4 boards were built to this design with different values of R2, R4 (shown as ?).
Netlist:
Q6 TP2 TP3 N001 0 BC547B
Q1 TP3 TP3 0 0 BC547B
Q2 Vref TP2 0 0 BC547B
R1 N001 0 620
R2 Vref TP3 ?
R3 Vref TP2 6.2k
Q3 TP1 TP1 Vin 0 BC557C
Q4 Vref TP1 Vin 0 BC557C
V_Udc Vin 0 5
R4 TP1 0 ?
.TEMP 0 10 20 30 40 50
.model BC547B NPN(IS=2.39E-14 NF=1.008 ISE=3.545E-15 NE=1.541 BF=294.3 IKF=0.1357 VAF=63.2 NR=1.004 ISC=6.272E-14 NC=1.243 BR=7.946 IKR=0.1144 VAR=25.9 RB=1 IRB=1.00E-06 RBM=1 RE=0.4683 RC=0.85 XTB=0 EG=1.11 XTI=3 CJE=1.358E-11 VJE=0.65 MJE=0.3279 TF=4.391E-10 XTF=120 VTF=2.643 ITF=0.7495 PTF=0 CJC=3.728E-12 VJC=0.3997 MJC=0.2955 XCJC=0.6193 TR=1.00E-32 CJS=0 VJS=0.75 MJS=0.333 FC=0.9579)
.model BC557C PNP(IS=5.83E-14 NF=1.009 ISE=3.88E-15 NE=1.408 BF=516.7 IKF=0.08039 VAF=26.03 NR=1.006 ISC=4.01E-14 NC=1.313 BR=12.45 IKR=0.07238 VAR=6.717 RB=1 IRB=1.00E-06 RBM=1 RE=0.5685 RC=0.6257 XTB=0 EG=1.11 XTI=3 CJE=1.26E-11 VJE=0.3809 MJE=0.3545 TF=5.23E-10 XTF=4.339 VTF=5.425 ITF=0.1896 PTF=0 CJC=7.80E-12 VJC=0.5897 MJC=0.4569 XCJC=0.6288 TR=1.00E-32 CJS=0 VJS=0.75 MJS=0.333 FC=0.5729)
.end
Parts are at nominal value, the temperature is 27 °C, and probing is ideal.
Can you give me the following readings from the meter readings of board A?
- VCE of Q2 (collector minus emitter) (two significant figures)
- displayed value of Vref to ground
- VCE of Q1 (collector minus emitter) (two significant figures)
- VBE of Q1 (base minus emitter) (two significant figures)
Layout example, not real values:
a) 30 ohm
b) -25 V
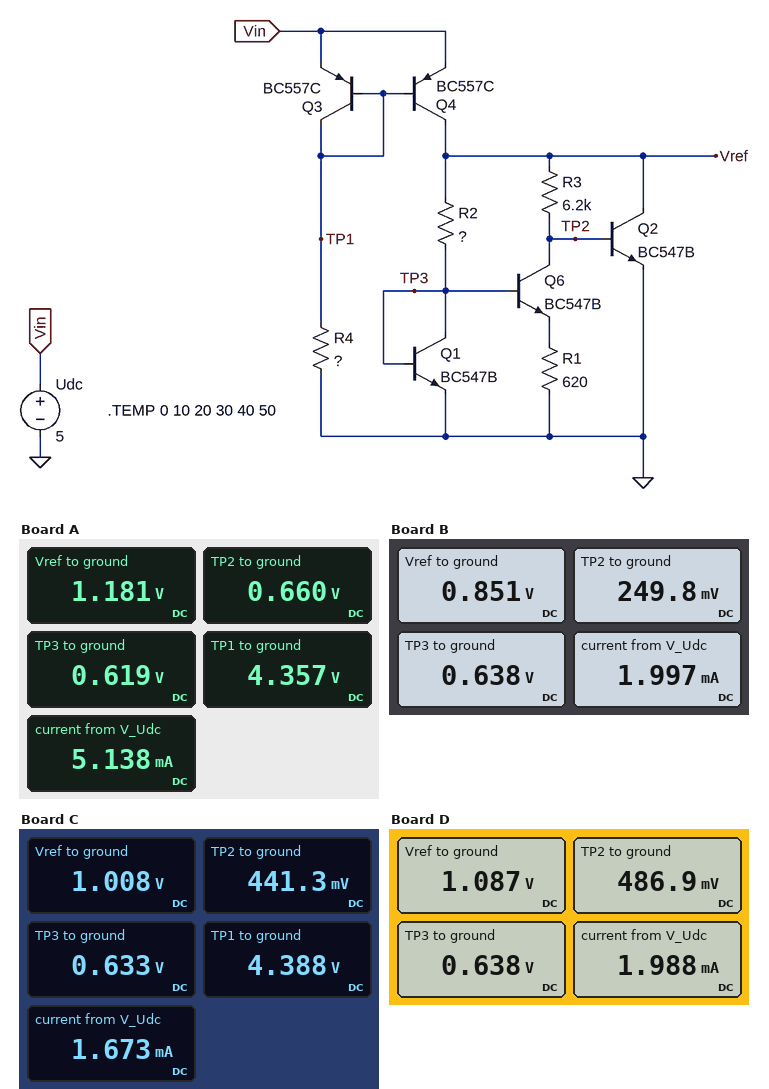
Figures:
a) 1.2 V
b) 1.181 V
c) 620 mV
d) 620 mV
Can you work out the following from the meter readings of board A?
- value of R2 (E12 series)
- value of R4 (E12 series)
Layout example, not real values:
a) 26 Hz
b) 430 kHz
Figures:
a) 1.2 kΩ
b) 1.8 kΩ
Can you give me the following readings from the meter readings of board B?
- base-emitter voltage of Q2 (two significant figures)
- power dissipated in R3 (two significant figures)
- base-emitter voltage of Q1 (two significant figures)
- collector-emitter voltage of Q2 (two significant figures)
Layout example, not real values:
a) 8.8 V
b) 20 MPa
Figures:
a) 250 mV
b) 58 µW
c) 640 mV
d) 850 mV
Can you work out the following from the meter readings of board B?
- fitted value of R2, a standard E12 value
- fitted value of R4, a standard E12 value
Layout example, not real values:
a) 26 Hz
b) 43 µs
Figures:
a) 220 Ω
b) 4.7 kΩ
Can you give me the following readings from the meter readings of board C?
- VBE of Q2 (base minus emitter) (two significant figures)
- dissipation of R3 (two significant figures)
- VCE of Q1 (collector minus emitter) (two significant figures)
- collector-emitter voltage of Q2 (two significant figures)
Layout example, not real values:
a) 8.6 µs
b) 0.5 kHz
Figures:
a) 440 mV
b) 52 µW
c) 630 mV
d) 1.0 V
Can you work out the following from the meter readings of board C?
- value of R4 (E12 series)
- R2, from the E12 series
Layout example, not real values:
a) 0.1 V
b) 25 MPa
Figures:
a) 5.6 kΩ
b) 470 Ω
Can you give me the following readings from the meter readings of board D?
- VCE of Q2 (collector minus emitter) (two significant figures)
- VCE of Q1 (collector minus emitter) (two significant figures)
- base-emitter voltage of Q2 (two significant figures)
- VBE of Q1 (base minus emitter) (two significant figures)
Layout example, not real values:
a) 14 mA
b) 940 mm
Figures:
a) 1.1 V
b) 640 mV
c) 490 mV
d) 640 mV
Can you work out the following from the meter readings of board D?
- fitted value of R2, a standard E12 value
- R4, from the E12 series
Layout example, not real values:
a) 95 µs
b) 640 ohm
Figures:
a) 470 Ω
b) 4.7 kΩ
